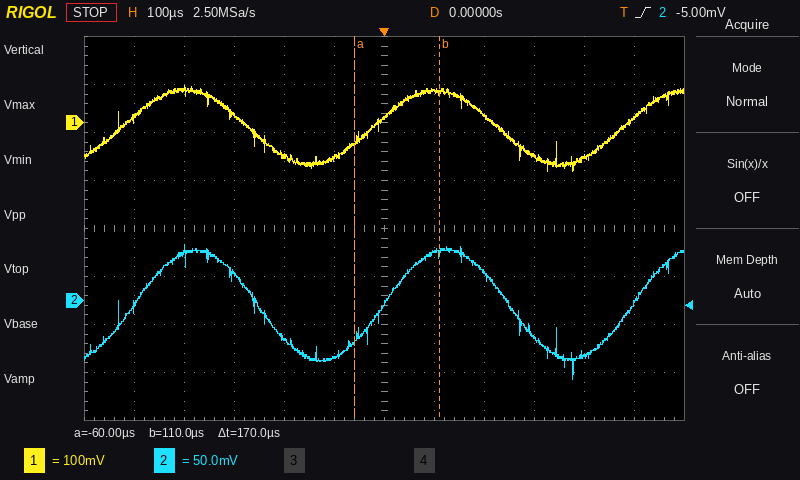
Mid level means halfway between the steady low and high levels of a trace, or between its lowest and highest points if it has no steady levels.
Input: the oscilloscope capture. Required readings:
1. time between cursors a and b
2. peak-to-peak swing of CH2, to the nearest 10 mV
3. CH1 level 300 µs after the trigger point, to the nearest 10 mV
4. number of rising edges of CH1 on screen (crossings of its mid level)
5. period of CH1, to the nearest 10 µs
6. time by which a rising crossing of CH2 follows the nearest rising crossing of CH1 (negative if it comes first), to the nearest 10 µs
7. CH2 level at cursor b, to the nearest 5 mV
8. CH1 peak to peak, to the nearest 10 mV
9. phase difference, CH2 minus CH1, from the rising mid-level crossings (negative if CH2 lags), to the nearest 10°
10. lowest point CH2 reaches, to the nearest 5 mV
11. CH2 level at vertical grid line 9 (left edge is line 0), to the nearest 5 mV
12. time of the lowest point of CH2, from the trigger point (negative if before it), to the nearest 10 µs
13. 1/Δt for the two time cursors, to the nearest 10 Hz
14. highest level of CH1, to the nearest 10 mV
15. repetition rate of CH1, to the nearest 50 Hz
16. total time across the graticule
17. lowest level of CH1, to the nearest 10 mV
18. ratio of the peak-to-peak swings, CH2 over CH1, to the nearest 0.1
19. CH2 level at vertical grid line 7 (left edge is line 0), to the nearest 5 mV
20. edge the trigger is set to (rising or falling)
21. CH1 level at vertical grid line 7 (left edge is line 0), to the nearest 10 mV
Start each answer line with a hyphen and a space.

- 170 µs
- 140 mV
- -70 mV
- 3
- 500 µs
- +20 µs
- 50 mV
- 180 mV
- -10°
- -80 mV
- -40 mV
- +380 µs
- 5.88 kHz
- 80 mV
- 2.00 kHz
- 1.2 ms
- -100 mV
- 0.8
- 50 mV
- rising
- 70 mV
